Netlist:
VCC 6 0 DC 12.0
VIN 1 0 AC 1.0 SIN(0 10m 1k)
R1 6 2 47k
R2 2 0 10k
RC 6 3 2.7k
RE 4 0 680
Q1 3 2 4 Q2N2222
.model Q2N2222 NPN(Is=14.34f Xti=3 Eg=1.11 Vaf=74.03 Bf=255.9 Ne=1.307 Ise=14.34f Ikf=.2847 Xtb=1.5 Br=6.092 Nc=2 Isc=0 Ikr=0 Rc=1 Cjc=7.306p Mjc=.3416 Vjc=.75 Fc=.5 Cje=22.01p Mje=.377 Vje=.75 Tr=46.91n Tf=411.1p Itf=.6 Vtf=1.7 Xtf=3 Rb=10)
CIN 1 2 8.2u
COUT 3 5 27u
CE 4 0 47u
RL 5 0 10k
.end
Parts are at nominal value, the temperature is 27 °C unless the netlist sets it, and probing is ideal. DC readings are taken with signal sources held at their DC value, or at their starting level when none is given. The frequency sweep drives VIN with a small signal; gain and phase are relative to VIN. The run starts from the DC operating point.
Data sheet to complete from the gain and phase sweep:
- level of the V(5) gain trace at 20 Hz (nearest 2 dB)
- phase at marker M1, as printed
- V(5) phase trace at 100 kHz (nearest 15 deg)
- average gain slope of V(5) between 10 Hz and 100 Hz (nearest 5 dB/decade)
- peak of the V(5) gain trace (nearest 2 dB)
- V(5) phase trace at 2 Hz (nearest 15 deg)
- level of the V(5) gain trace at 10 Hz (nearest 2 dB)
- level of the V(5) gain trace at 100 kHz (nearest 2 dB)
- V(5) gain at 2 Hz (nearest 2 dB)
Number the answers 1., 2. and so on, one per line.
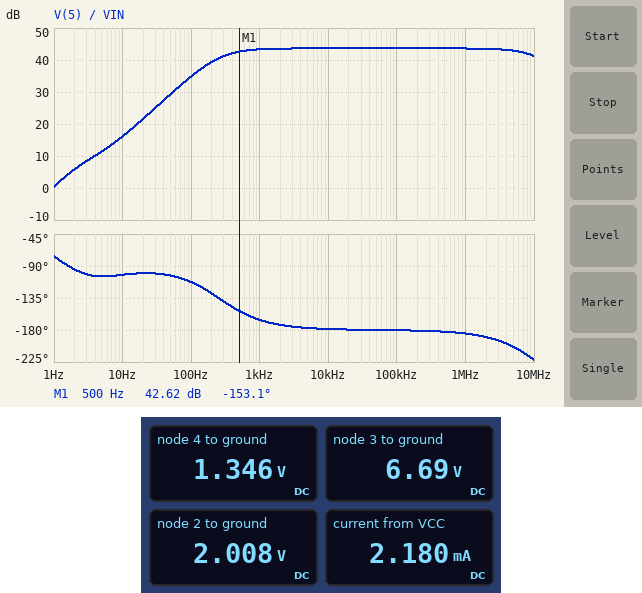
1. 22 dB
2. -153.1 deg
3. -180 deg
4. 20 dB/decade
5. 44 dB
6. -90 deg
7. 16 dB
8. 44 dB
9. 6 dB
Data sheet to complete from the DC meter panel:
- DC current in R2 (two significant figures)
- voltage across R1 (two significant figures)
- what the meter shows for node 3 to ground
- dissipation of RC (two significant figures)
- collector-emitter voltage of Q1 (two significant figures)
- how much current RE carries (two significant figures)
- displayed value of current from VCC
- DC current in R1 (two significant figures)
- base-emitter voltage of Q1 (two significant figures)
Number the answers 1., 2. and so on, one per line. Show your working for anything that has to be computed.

1. (2.008 V) / 10 kΩ = 200 µA
2. 12 V - 2.008 V = 10 V
3. 6.69 V
4. (12 V - 6.69 V)^2 / 2.7 kΩ = 10 mW
5. 6.69 V - 1.346 V = 5.3 V
6. (1.346 V) / 680 Ω = 2.0 mA
7. 2.180 mA
8. (12 V - 2.008 V) / 47 kΩ = 210 µA
9. 2.008 V - 1.346 V = 660 mV
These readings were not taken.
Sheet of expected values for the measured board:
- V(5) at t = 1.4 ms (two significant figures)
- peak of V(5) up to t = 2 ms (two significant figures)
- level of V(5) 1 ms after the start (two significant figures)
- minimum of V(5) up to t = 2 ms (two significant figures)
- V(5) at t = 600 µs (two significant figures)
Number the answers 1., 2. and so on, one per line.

1. -420 mV
2. 1.4 V
3. -200 mV
4. -1.5 V
5. 1.1 V
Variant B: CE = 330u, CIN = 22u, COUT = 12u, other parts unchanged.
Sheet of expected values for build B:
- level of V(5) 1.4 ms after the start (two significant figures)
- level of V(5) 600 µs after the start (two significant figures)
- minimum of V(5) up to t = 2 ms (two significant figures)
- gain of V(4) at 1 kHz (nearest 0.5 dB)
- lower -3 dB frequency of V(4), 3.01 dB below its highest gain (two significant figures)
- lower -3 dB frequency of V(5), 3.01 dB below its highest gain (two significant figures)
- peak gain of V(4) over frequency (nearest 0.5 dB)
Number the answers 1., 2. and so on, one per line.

1. -830 mV
2. 900 mV
3. -1.7 V
4. -29.0 dB
5. 830 mHz
6. 38 Hz
7. -1.0 dB
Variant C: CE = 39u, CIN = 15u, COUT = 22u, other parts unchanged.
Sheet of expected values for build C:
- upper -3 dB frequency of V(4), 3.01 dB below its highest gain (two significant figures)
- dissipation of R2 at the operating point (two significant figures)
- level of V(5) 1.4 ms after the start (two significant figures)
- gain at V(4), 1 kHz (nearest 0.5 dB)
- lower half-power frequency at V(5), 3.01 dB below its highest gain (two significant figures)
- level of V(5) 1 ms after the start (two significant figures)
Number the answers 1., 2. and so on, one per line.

1. 310 Hz
2. 400 µW
3. -360 mV
4. -11.0 dB
5. 300 Hz
6. -270 mV
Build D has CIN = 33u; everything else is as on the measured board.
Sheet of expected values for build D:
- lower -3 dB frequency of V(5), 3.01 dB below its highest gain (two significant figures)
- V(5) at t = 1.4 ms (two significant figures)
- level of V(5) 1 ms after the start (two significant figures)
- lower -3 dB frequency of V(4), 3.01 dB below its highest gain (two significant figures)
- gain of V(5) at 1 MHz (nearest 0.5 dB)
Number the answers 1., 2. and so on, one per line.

1. 250 Hz
2. -430 mV
3. -190 mV
4. 620 mHz
5. 43.5 dB
